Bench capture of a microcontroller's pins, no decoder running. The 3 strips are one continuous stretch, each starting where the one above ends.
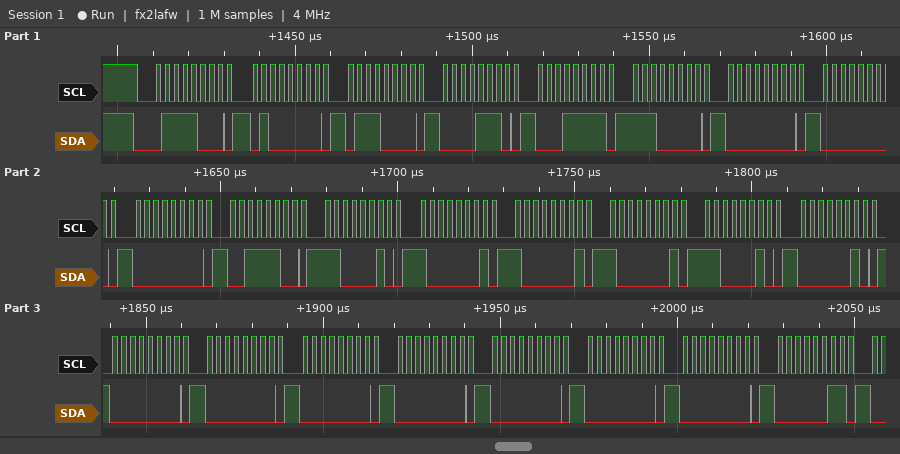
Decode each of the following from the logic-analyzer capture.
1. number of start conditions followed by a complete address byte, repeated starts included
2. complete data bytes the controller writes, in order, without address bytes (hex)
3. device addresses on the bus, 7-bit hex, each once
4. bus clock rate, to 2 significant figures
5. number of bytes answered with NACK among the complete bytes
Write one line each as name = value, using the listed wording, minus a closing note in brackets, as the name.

number of start conditions followed by a complete address byte, repeated starts included = 1
complete data bytes the controller writes, in order, without address bytes = 40 70 0E 1F E0 00 00 00 3C C2 81 81 81 C2 02 00 00 00 00 00 00 00 03
device addresses on the bus, 7-bit hex, each once = 0x3C
bus clock rate, to 2 significant figures = 400 kHz
number of bytes answered with NACK among the complete bytes = 0
